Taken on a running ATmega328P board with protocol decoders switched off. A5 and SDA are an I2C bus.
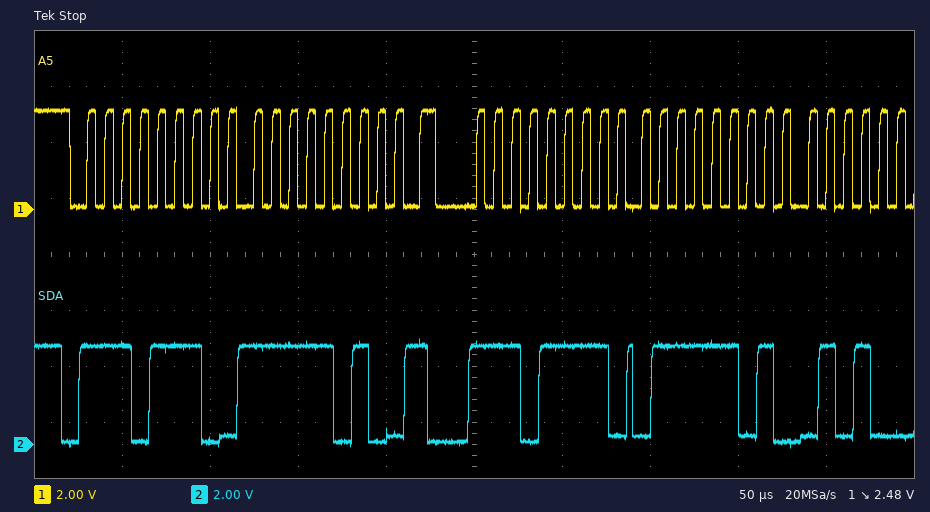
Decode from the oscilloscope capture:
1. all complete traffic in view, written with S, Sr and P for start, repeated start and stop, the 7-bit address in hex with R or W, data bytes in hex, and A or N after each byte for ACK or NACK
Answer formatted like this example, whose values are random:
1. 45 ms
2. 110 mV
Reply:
1. S 77W A FA A Sr 77R A 7D A
